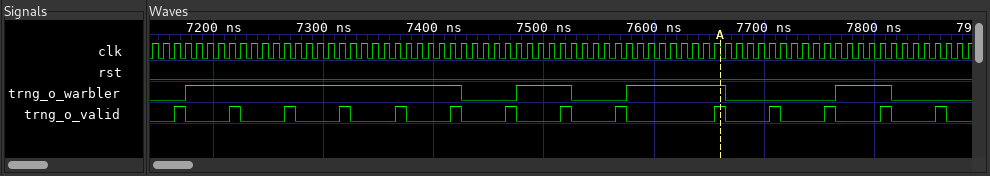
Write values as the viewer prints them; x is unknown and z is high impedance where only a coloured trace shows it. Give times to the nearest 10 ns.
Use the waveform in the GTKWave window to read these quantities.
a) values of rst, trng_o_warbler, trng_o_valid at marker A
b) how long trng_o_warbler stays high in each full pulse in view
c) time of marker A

rst=0, trng_o_warbler=1, trng_o_valid=1
250 ns, 50 ns, 90 ns, 50 ns
7660 ns
